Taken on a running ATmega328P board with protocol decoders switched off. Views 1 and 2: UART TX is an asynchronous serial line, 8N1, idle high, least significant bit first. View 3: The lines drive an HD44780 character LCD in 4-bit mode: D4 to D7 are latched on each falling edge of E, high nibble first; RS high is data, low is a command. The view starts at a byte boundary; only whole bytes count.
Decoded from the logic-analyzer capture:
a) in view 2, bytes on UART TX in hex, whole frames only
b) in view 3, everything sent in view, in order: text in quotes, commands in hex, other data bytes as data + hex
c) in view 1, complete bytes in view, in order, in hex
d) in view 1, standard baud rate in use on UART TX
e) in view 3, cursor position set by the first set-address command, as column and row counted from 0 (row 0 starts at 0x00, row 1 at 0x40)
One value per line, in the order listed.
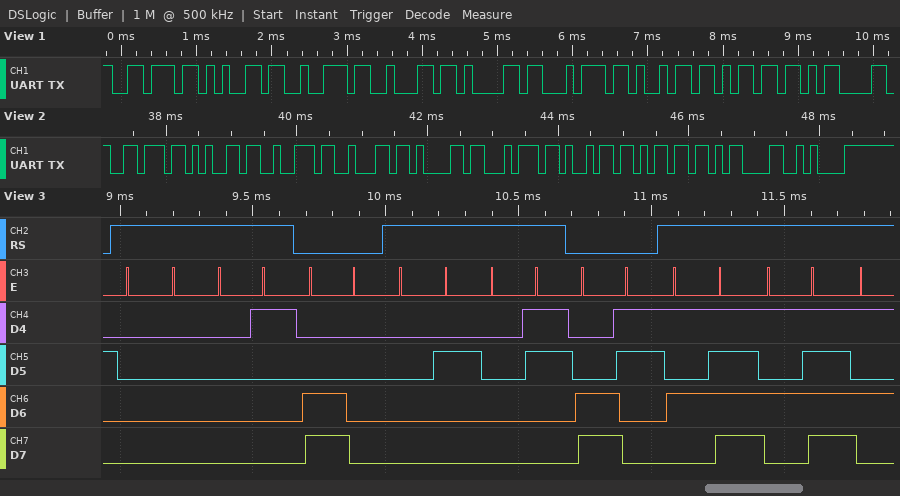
0x76 0x65 0x72 0x62 0x61 0x74 0x69 0x6D 0x0D 0x0A
data 00 01 0xC0 data 02 03 0xC3 "__"
0x76 0x65 0x72 0x62 0x61 0x74 0x69 0x6D 0x0D
9600 baud
column 0, row 1
